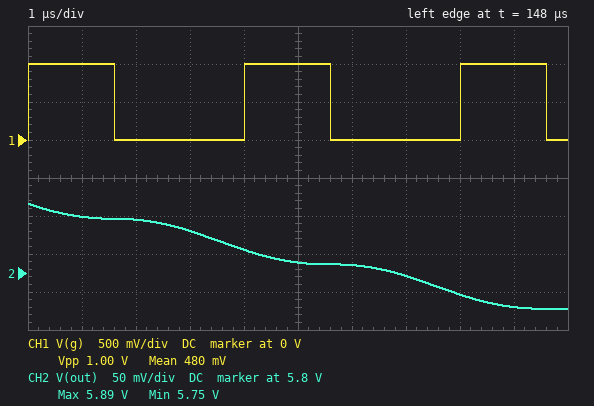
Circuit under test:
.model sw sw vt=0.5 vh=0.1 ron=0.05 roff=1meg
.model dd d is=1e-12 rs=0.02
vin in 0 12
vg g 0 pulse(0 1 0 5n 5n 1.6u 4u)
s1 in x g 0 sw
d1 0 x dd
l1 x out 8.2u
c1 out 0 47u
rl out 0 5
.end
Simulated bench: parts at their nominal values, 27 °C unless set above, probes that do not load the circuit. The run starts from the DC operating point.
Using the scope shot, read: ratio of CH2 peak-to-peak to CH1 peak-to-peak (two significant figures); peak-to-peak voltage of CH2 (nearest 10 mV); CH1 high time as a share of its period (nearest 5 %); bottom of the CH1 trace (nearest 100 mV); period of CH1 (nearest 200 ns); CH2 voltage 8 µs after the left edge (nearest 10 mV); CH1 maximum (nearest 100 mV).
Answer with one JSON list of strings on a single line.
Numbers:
["0.14", "140 mV", "40 %", "0 V", "4.0 µs", "5.77 V", "1.0 V"]
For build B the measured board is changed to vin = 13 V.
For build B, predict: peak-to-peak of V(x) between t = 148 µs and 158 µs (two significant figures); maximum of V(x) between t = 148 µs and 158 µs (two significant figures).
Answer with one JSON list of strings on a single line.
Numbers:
["14 V", "13 V"]
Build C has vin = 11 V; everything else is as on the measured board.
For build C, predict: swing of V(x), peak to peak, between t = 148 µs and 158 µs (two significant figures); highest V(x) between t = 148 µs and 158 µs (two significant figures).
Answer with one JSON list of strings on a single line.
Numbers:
["12 V", "11 V"]
